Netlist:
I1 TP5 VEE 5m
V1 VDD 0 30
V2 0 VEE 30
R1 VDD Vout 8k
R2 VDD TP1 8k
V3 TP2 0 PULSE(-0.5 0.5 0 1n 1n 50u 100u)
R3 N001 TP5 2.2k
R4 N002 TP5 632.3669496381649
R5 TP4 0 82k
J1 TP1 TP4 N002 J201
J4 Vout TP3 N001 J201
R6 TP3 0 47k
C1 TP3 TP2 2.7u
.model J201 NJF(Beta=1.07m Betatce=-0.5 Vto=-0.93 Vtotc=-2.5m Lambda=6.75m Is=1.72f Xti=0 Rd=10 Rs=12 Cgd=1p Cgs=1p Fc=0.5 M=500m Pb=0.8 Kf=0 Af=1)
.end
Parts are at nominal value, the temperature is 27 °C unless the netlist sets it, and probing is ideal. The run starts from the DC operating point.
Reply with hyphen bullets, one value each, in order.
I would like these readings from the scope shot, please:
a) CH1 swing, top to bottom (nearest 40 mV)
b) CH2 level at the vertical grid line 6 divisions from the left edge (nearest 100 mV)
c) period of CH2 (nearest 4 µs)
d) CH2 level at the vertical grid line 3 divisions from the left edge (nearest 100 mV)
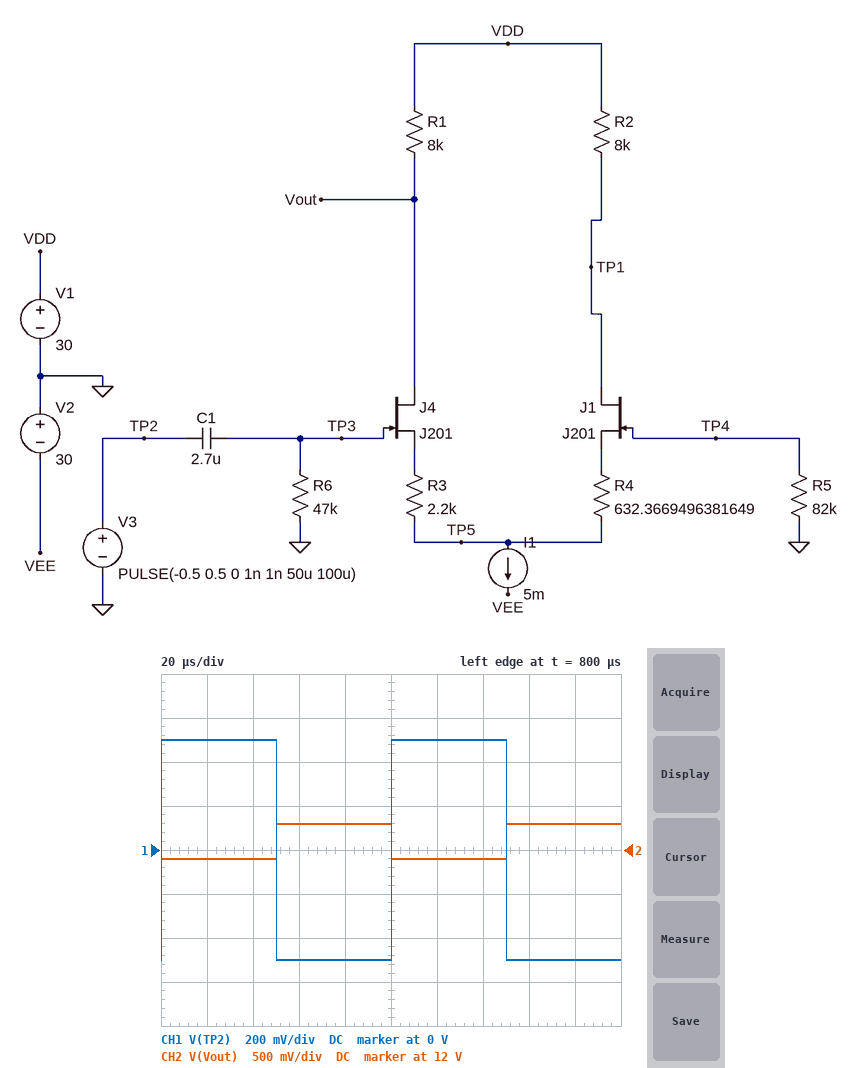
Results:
- 1.00 V
- 11.9 V
- 100 µs
- 12.3 V
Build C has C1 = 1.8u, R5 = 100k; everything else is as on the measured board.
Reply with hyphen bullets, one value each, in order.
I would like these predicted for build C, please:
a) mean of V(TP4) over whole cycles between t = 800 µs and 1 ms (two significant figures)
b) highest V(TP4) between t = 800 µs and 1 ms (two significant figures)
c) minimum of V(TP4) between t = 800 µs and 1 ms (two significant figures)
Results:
- -2.6 V
- -2.2 V
- -3.0 V
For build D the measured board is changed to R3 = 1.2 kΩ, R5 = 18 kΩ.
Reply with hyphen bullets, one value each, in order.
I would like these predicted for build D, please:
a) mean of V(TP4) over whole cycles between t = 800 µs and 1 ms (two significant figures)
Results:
- -460 mV
